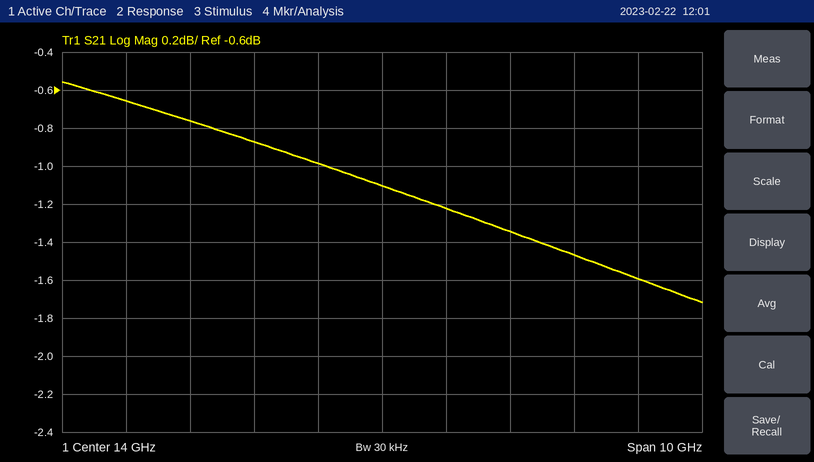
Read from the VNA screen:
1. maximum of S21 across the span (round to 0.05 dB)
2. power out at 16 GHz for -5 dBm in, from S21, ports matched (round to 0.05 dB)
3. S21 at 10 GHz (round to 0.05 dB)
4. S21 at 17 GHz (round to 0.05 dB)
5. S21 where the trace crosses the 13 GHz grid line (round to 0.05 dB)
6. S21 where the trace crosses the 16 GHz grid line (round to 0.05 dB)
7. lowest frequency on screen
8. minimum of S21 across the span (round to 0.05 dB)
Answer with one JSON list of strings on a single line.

["-0.55 dB", "-6.35 dBm", "-0.65 dB", "-1.45 dB", "-1.00 dB", "-1.35 dB", "9 GHz", "-1.70 dB"]
